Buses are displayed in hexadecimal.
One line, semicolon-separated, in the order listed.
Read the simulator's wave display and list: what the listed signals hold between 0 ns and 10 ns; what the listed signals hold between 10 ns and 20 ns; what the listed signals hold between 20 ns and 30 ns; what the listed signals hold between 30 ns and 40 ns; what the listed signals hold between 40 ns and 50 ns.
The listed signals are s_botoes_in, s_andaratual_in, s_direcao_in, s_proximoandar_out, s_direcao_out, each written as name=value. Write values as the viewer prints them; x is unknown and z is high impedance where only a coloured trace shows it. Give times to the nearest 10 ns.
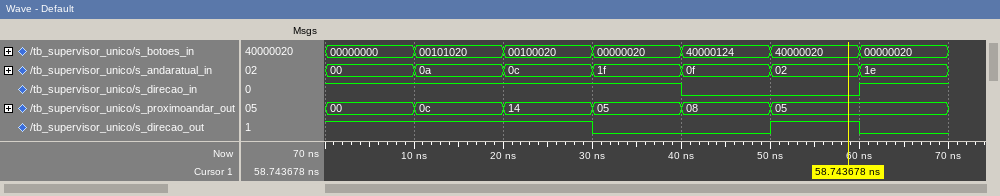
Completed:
s_botoes_in=00000000, s_andaratual_in=00, s_direcao_in=1, s_proximoandar_out=00, s_direcao_out=1; s_botoes_in=00101020, s_andaratual_in=0a, s_direcao_in=1, s_proximoandar_out=0c, s_direcao_out=1; s_botoes_in=00100020, s_andaratual_in=0c, s_direcao_in=1, s_proximoandar_out=14, s_direcao_out=1; s_botoes_in=00000020, s_andaratual_in=1f, s_direcao_in=1, s_proximoandar_out=05, s_direcao_out=0; s_botoes_in=40000124, s_andaratual_in=0f, s_direcao_in=0, s_proximoandar_out=08, s_direcao_out=0
